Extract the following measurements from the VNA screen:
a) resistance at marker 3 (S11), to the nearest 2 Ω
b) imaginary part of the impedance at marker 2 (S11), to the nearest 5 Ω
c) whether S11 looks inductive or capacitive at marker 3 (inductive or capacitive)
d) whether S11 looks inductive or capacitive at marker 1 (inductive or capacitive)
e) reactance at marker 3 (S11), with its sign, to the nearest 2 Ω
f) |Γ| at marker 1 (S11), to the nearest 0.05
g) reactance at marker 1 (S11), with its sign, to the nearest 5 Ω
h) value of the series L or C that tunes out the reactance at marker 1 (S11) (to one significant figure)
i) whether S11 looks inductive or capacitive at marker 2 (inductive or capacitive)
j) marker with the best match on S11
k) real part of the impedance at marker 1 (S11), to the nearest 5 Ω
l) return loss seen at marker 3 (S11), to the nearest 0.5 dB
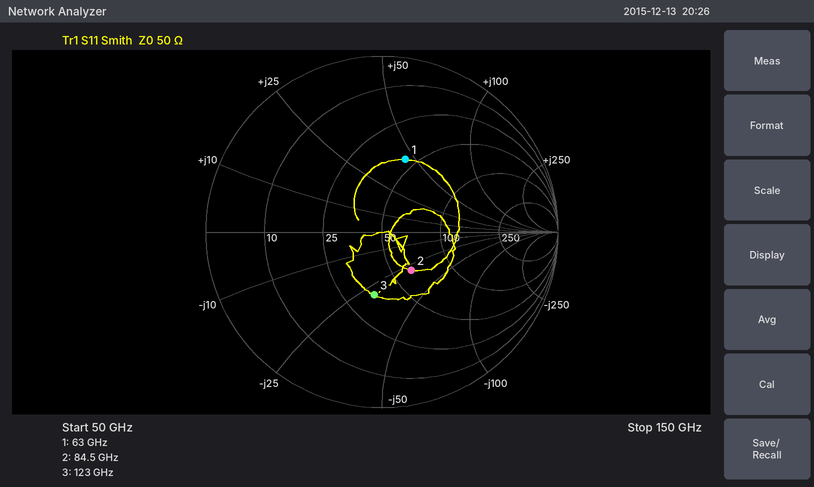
36 Ω
-30 Ω
capacitive
inductive
-30 Ω
0.45
+45 Ω
60 fF
capacitive
marker 2
45 Ω
9.0 dB
